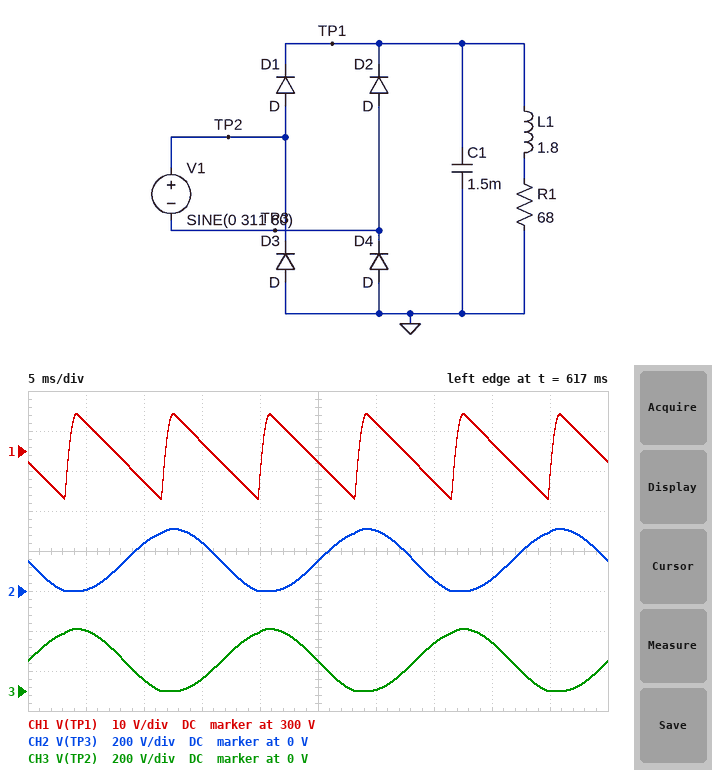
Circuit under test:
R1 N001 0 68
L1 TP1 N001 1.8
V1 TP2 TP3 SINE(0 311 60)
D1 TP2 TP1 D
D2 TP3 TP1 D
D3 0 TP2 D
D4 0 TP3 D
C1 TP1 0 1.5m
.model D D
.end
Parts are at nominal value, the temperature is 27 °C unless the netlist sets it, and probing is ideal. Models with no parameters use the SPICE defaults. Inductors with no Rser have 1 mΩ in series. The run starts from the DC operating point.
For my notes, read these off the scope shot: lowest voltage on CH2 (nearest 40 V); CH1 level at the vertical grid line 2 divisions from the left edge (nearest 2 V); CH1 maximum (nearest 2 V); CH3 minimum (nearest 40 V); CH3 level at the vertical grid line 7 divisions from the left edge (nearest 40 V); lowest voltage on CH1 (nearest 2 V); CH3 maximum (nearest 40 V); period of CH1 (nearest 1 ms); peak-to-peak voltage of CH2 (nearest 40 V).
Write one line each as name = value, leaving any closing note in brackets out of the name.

lowest voltage on CH2 = 0 V
CH1 level at the vertical grid line 2 divisions from the left edge = 292 V
CH1 maximum = 310 V
CH3 minimum = 0 V
CH3 level at the vertical grid line 7 divisions from the left edge = 240 V
lowest voltage on CH1 = 288 V
CH3 maximum = 320 V
period of CH1 = 8 ms
peak-to-peak voltage of CH2 = 320 V
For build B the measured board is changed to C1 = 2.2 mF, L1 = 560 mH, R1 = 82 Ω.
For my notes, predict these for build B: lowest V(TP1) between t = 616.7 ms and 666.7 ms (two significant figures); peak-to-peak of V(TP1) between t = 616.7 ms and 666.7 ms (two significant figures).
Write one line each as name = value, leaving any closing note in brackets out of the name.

lowest V(TP1) between t = 616.7 ms and 666.7 ms = 300 V
peak-to-peak of V(TP1) between t = 616.7 ms and 666.7 ms = 13 V
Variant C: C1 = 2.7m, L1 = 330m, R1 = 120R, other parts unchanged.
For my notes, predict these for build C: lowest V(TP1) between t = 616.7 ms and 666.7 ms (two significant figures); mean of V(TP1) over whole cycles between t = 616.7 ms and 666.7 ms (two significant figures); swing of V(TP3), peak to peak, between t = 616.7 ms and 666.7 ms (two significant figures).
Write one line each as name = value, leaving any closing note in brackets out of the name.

lowest V(TP1) between t = 616.7 ms and 666.7 ms = 300 V
mean of V(TP1) over whole cycles between t = 616.7 ms and 666.7 ms = 310 V
swing of V(TP3), peak to peak, between t = 616.7 ms and 666.7 ms = 310 V
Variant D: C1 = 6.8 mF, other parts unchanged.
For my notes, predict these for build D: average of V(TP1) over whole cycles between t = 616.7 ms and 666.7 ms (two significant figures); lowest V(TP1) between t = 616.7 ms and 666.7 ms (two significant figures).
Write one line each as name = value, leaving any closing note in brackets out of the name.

average of V(TP1) over whole cycles between t = 616.7 ms and 666.7 ms = 310 V
lowest V(TP1) between t = 616.7 ms and 666.7 ms = 300 V
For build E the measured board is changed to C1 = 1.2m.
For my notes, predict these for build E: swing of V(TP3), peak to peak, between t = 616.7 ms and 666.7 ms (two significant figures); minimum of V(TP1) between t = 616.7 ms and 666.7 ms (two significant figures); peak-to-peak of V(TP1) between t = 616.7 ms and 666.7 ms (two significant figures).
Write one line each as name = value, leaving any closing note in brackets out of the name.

swing of V(TP3), peak to peak, between t = 616.7 ms and 666.7 ms = 310 V
minimum of V(TP1) between t = 616.7 ms and 666.7 ms = 280 V
peak-to-peak of V(TP1) between t = 616.7 ms and 666.7 ms = 26 V
